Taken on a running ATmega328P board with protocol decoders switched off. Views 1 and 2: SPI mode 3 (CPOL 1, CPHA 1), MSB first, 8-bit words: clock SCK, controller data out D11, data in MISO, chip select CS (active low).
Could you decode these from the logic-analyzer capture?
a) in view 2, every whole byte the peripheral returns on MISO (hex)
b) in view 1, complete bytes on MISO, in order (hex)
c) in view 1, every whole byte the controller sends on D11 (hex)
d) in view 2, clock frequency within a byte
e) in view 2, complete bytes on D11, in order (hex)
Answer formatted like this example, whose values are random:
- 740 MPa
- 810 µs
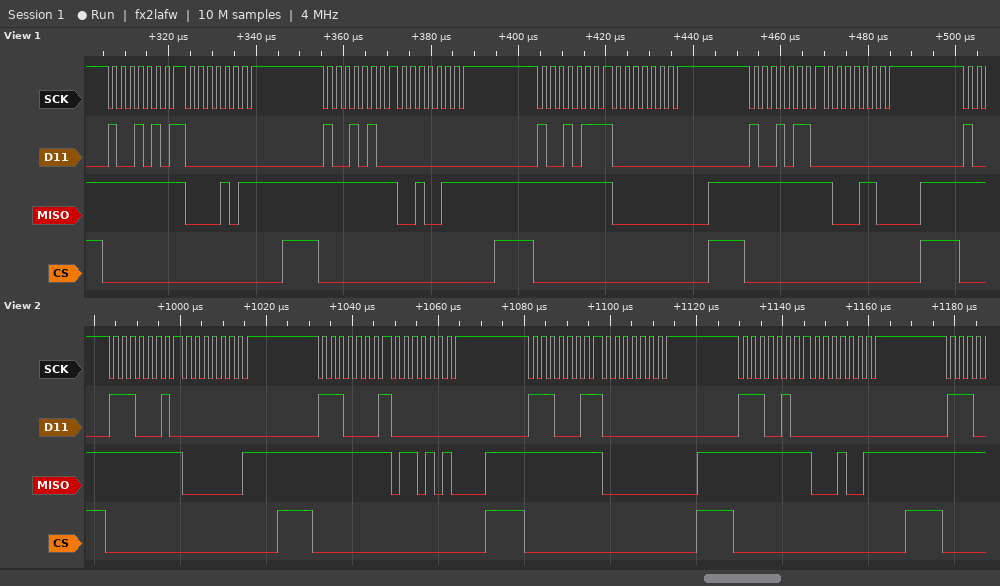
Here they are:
- FF 01 FF 6A FF 00 FF 13
- FF 0B FF 27 FF 00 FF 8C
- 95 00 94 00 97 00 96 00
- 500 kHz
- E2 00 E1 00 E3 00 E4 00
